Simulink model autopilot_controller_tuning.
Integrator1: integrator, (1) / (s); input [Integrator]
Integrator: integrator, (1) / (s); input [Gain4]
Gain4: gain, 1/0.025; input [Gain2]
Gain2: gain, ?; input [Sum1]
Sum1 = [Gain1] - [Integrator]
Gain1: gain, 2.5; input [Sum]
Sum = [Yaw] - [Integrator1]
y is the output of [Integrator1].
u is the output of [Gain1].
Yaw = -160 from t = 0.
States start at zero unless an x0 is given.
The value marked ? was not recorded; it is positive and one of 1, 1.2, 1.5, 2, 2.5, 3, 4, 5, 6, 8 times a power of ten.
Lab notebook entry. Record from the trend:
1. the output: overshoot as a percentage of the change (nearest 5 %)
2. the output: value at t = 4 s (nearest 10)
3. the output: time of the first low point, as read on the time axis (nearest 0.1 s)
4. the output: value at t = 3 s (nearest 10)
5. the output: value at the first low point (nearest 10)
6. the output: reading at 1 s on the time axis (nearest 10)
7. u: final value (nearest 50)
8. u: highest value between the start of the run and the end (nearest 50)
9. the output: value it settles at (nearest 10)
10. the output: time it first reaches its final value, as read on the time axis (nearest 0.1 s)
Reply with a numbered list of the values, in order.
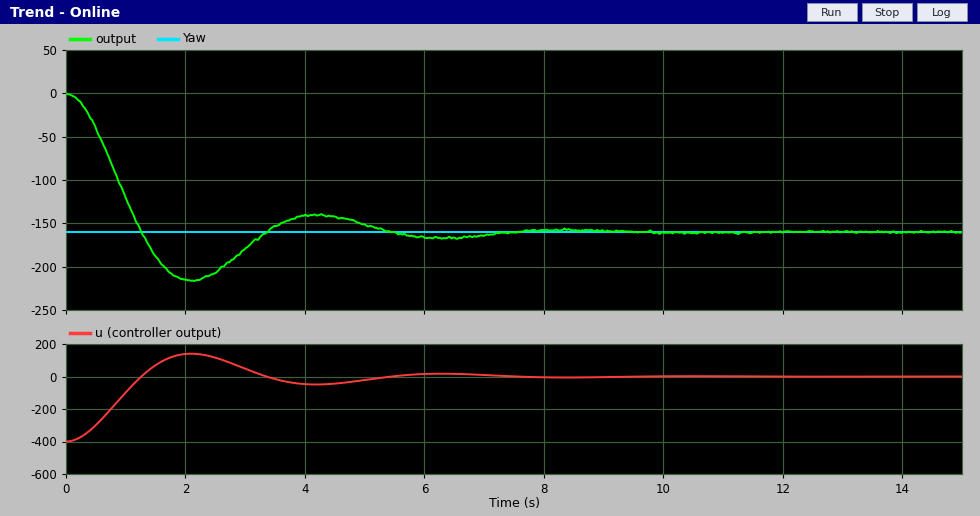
1. 35 %
2. -140
3. 2.1 s
4. -180
5. -220
6. -120
7. 0
8. 150
9. -160
10. 1.3 s
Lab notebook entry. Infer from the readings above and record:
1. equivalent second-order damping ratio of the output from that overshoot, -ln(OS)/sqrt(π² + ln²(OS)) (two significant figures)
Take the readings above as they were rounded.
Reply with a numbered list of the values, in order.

1. 0.32
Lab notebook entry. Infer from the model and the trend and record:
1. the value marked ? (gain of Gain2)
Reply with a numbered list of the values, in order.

1. 0.025
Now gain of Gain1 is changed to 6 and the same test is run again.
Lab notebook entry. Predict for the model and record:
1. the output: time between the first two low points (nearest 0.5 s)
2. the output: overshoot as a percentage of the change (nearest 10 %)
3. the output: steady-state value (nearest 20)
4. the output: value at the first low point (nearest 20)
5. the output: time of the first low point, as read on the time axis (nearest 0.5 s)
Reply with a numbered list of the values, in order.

1. 2.5 s
2. 50 %
3. -160
4. -240
5. 1.5 s
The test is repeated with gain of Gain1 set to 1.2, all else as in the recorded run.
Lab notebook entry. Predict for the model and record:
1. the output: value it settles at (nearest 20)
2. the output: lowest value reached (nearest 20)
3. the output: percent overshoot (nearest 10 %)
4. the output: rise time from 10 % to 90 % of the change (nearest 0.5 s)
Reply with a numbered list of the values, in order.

1. -160
2. -200
3. 20 %
4. 1.5 s
